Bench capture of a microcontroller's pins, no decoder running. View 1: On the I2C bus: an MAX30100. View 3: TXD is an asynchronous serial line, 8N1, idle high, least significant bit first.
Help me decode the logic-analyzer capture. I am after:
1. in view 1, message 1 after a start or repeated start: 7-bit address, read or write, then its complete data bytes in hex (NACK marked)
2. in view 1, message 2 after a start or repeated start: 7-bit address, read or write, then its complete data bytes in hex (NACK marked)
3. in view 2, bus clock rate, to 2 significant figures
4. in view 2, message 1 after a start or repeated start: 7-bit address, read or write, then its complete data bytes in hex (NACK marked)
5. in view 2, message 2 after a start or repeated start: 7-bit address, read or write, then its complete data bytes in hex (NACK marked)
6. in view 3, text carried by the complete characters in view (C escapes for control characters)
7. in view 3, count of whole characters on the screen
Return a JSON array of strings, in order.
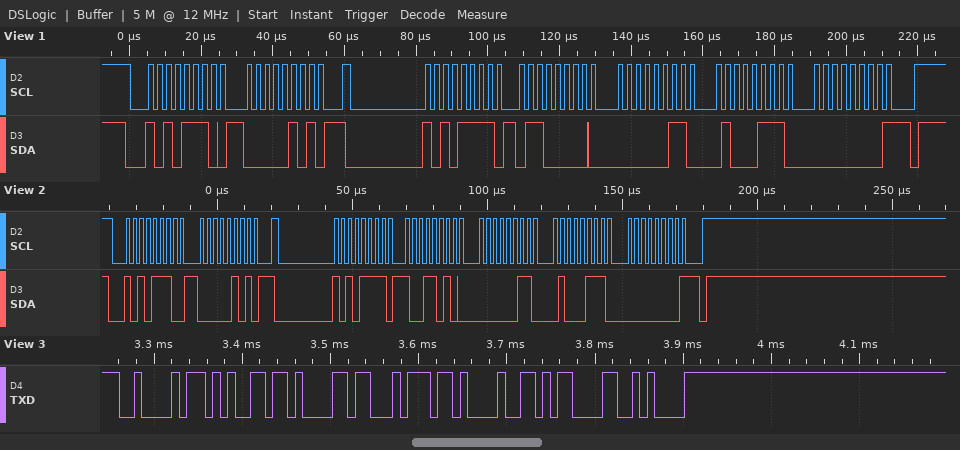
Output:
["0x57 write: 05", "0x57 read: 60 03 47 00 NACK", "400 kHz", "0x57 write: 05", "0x57 read: 9A 03 47 00 NACK", "\"Beat!\\r\\n\"", "7"]
